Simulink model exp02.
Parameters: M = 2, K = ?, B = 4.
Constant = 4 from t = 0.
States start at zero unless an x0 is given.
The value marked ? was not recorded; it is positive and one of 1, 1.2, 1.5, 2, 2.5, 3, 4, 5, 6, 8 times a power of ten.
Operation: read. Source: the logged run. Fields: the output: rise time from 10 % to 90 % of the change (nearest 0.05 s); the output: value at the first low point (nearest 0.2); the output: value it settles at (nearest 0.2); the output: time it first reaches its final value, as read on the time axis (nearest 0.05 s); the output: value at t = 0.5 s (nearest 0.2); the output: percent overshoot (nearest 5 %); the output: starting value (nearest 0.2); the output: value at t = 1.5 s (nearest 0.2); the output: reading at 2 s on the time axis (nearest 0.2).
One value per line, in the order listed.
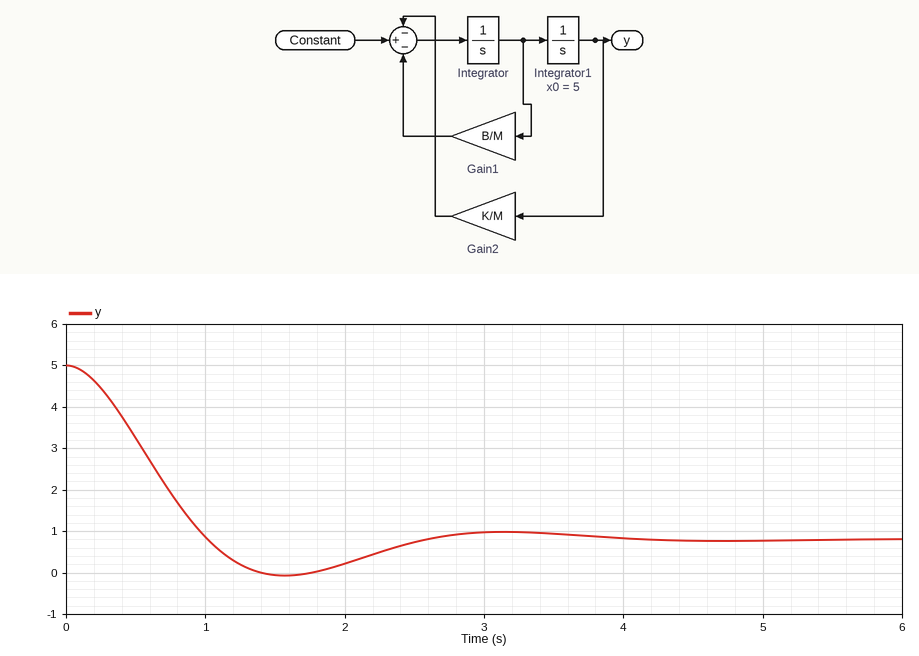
0.70 s
0.0
0.8
1.00 s
3.2
20 %
5.0
0.0
0.2
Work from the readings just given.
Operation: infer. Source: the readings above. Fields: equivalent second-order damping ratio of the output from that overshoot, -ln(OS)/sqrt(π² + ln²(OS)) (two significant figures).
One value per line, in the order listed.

0.46
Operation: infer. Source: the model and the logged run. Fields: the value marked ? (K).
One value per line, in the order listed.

10
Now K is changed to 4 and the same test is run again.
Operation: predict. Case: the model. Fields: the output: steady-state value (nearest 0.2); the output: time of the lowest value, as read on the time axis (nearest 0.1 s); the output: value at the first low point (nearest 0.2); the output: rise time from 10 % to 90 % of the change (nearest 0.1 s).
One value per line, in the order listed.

2.0
3.1 s
1.8
1.5 s
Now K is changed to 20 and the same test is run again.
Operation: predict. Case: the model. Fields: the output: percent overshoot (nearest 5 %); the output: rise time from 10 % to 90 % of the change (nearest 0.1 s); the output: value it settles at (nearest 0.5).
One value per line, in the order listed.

35 %
0.4 s
0.5
